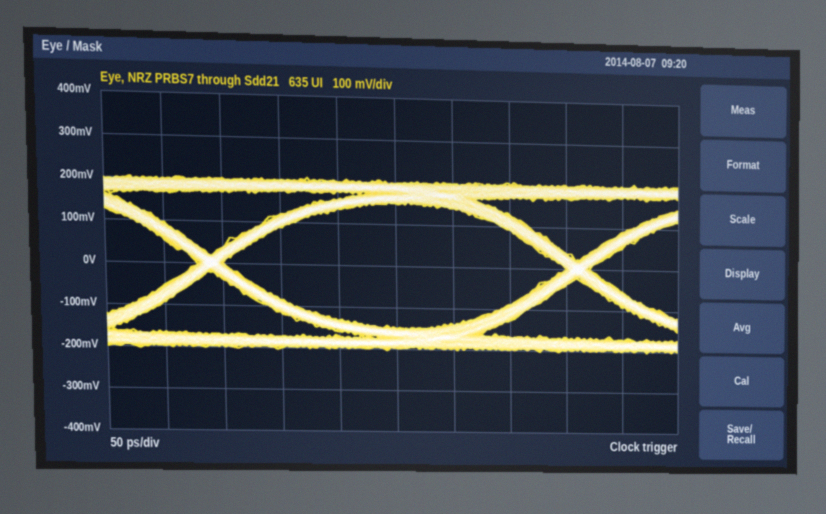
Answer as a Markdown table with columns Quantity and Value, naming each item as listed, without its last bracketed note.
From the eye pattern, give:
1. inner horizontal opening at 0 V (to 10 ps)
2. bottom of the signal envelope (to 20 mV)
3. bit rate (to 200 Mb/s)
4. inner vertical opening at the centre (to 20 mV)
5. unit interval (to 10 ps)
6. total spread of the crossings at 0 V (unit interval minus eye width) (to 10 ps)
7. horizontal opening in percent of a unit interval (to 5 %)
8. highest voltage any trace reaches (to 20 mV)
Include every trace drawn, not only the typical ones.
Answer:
| Quantity | Value |
|---|---|
| inner horizontal opening at 0 V | 300 ps |
| bottom of the signal envelope | -200 mV |
| bit rate | 3.2 Gb/s |
| inner vertical opening at the centre | 300 mV |
| unit interval | 320 ps |
| total spread of the crossings at 0 V (unit interval minus eye width) | 20 ps |
| horizontal opening in percent of a unit interval | 95 % |
| highest voltage any trace reaches | 200 mV |
